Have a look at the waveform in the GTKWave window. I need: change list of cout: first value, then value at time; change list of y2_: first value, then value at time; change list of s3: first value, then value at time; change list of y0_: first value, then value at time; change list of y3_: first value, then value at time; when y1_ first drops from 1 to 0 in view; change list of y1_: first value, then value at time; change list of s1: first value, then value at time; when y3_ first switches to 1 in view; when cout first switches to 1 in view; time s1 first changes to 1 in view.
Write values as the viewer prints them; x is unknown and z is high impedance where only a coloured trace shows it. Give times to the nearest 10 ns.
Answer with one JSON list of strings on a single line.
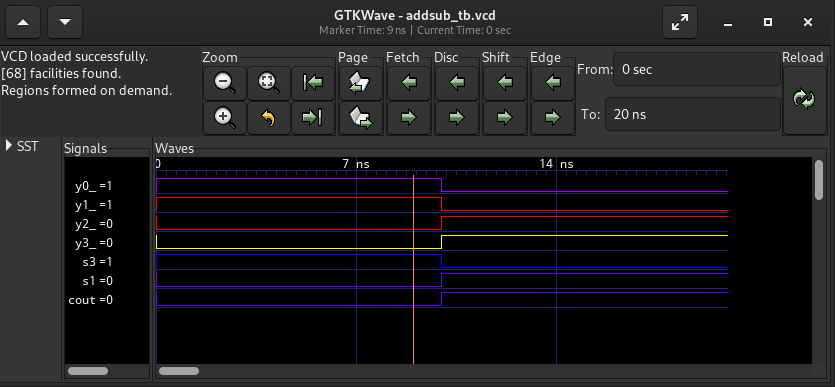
["0, 1 at 10 ns", "0, 1 at 10 ns", "1, 0 at 10 ns", "1, 0 at 10 ns", "0, 1 at 10 ns", "10 ns", "1, 0 at 10 ns", "0, 1 at 10 ns", "10 ns", "10 ns", "10 ns"]
